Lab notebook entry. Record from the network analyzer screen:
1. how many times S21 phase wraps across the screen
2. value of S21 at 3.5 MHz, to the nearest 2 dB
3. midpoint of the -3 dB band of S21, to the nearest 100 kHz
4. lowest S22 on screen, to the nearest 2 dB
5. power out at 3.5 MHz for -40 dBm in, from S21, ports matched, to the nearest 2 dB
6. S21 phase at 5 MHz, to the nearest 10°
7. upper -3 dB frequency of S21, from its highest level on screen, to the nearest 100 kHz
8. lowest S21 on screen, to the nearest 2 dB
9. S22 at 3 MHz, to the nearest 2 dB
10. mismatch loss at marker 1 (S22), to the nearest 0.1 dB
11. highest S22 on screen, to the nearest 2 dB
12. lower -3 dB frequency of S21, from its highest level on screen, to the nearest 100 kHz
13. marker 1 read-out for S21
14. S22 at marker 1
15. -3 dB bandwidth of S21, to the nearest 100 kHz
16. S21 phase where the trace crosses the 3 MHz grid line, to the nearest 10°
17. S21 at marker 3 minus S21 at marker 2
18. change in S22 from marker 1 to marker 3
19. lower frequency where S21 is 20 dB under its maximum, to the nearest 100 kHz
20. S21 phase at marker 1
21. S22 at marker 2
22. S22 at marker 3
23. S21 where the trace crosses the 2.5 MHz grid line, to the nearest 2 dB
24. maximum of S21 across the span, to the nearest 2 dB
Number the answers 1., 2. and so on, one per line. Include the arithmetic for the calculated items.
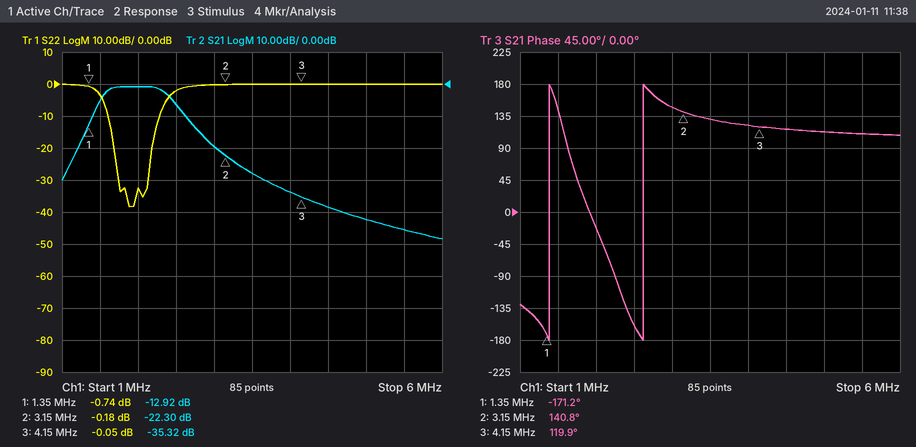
1. 2
2. -28 dB
3. 2.0 MHz
4. -38 dB
5. -40 dBm + (-28 dB) = -68 dBm
6. 110°
7. 2.4 MHz
8. -48 dB
9. 0 dB
10. −10 log10(1 − 10^(-0.74/10)) ≈ 8.1 dB
11. 0 dB
12. 1.5 MHz
13. -12.92 dB
14. -0.74 dB
15. 2.4 MHz − 1.5 MHz = 900 kHz
16. 150°
17. -35.32 − (-22.3) = -13.02 dB
18. -0.05 − (-0.74) = 0.69 dB
19. 1.2 MHz
20. -171.2°
21. -0.18 dB
22. -0.05 dB
23. -6 dB
24. 0 dB
